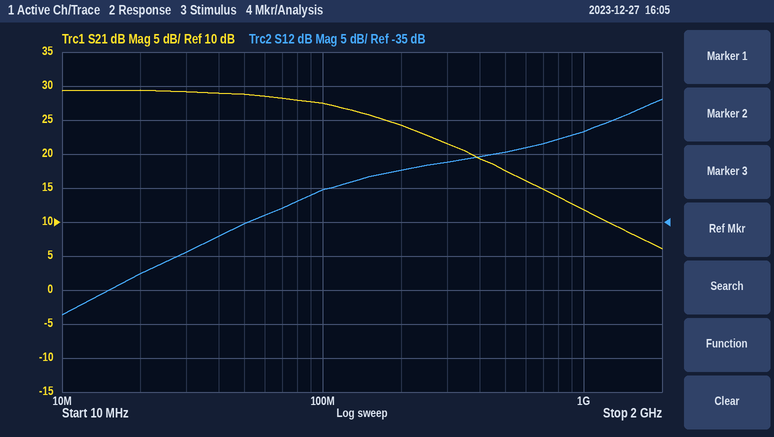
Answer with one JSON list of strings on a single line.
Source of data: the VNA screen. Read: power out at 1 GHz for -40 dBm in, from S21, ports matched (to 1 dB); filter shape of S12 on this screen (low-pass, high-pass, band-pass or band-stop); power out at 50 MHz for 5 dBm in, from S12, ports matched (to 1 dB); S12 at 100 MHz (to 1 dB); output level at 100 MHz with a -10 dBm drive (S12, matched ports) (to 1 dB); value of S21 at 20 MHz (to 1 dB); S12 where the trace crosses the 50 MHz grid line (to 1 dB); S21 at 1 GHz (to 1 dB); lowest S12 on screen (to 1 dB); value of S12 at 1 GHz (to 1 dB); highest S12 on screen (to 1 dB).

["-28 dBm", "high-pass", "-30 dBm", "-30 dB", "-40 dBm", "29 dB", "-35 dB", "12 dB", "-49 dB", "-22 dB", "-17 dB"]
